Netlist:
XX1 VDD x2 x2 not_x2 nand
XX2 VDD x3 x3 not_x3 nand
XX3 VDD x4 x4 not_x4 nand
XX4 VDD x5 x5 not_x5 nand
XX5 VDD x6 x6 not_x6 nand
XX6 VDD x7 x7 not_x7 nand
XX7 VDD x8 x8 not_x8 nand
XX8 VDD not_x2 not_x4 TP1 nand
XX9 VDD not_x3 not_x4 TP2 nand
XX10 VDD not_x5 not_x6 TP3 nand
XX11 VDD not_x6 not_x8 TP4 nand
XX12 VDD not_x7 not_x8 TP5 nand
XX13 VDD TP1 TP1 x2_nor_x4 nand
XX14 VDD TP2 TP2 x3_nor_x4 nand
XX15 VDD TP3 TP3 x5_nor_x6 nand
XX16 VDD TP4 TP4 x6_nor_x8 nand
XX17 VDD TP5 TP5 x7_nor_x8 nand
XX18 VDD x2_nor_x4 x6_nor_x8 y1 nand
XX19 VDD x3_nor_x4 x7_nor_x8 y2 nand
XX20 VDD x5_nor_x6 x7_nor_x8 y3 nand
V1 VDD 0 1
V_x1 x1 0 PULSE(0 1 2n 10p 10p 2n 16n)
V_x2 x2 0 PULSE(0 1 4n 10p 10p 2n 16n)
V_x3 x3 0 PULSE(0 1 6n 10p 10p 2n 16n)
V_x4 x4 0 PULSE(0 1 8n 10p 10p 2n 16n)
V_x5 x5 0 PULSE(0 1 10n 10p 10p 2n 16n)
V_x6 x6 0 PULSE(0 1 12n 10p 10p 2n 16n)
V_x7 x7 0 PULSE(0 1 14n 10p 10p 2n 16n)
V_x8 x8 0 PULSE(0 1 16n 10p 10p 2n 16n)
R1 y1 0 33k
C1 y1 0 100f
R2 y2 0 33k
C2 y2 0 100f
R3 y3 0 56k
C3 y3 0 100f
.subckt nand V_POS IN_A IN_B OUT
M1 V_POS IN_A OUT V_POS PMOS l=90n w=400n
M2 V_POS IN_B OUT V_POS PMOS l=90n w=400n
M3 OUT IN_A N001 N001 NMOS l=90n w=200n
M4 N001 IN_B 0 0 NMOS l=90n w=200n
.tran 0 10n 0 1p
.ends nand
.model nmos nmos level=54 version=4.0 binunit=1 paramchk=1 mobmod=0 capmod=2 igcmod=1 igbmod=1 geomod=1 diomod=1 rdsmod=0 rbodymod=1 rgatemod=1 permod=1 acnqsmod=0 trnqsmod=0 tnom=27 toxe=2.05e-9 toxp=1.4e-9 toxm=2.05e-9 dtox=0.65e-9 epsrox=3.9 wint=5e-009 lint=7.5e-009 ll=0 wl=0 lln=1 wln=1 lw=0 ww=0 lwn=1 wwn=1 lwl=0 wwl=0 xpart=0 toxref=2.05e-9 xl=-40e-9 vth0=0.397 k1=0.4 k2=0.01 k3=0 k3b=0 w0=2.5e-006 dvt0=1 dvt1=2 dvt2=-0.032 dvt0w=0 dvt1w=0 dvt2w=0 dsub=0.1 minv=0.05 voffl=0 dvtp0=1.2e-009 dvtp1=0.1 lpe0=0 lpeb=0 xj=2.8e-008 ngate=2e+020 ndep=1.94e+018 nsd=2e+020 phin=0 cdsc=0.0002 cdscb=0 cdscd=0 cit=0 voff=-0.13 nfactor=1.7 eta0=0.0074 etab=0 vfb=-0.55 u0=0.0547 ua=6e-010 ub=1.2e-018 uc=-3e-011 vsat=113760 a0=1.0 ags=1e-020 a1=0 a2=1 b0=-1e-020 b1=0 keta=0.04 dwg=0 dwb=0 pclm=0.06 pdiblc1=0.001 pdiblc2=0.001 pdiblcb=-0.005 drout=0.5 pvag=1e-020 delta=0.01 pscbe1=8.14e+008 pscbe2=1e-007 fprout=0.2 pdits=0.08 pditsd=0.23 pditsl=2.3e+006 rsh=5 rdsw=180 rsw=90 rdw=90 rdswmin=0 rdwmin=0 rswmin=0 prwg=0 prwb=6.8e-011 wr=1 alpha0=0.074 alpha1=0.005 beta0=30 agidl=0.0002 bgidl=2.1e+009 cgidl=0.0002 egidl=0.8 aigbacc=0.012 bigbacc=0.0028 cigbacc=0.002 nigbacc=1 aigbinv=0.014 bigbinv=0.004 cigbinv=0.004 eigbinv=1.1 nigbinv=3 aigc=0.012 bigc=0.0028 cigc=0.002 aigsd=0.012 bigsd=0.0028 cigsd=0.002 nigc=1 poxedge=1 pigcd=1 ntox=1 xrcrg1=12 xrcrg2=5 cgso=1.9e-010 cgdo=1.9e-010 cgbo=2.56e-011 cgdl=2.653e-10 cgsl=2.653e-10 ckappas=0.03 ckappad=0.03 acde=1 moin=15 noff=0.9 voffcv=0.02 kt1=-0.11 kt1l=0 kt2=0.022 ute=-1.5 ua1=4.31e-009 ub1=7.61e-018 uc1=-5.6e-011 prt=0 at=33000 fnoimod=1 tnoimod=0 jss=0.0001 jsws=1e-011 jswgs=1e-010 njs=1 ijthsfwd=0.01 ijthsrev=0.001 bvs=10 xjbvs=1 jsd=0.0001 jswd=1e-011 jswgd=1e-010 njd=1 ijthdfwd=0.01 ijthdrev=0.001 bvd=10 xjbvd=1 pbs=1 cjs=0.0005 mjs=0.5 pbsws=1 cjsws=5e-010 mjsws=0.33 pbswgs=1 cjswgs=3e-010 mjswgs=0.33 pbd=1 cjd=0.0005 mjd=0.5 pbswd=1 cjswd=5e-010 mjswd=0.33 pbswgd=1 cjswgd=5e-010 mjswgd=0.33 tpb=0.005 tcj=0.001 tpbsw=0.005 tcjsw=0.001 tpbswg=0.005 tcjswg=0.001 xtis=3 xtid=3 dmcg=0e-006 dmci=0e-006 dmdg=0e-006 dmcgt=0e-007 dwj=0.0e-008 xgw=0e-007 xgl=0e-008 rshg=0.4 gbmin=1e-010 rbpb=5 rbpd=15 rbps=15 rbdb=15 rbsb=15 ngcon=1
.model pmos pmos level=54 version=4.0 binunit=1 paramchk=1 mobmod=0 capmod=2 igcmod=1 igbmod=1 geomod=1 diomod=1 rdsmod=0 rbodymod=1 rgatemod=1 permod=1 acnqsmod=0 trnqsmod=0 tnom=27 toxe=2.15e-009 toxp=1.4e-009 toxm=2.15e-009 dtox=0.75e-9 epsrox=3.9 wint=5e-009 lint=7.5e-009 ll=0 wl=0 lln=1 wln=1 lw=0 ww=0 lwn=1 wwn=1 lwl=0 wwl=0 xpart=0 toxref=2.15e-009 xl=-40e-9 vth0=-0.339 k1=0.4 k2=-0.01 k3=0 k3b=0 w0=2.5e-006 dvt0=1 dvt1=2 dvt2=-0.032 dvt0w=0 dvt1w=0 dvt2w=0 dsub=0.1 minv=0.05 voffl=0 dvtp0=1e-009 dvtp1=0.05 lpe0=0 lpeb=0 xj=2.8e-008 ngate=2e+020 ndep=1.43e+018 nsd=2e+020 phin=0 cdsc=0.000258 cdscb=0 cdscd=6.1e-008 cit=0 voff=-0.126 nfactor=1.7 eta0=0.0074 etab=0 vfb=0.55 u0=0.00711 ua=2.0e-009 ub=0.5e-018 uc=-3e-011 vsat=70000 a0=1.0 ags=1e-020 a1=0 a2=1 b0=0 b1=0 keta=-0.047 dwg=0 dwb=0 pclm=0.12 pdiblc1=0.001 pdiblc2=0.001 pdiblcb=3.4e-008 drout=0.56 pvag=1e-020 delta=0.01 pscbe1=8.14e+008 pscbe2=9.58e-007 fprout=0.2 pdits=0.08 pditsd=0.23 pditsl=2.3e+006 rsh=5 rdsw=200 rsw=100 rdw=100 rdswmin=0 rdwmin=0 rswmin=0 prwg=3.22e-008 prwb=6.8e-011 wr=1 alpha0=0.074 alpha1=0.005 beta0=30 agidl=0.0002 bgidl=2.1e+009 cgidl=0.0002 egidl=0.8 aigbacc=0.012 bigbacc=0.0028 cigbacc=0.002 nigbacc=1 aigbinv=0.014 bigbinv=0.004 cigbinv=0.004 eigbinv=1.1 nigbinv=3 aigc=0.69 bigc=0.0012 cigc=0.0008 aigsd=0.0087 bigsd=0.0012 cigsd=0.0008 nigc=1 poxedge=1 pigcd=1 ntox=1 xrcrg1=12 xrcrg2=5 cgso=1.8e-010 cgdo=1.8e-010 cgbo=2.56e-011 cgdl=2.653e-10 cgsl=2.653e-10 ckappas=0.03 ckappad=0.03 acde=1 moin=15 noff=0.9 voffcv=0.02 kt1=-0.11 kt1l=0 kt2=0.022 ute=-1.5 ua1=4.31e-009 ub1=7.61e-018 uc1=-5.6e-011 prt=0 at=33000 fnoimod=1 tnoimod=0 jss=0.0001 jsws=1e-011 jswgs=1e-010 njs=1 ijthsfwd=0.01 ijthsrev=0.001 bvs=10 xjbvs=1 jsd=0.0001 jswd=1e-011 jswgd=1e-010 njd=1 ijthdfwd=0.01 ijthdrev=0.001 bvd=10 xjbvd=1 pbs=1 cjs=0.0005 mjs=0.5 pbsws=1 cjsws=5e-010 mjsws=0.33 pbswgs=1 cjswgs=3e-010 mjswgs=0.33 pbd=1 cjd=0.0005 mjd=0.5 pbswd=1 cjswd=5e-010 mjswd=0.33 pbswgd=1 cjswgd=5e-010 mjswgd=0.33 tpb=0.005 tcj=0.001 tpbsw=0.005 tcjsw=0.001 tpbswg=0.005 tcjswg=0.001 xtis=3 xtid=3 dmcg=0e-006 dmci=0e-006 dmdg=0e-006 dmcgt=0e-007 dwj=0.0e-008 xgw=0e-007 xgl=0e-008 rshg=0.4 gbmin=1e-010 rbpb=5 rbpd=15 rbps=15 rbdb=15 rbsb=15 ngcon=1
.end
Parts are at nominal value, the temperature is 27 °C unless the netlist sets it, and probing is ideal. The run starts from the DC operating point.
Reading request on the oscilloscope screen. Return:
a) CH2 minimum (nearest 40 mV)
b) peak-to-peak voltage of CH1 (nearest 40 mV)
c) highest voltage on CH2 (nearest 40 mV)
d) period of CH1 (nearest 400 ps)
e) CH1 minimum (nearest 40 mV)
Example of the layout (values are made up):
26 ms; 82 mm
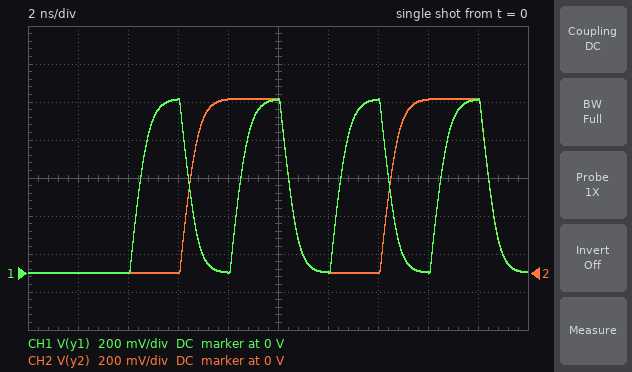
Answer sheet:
0 V; 920 mV; 920 mV; 4.0 ns; 0 V
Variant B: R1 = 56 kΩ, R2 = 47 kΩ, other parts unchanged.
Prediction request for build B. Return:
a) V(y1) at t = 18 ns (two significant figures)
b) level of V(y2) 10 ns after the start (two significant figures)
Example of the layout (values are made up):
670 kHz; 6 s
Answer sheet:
950 mV; 940 mV
